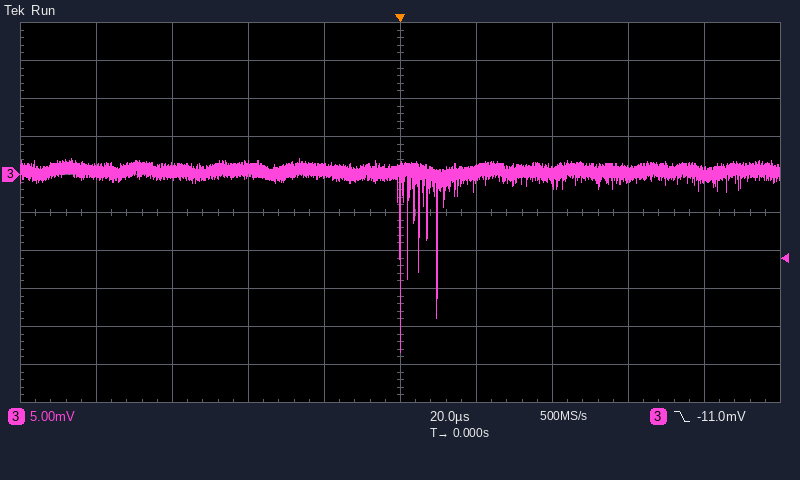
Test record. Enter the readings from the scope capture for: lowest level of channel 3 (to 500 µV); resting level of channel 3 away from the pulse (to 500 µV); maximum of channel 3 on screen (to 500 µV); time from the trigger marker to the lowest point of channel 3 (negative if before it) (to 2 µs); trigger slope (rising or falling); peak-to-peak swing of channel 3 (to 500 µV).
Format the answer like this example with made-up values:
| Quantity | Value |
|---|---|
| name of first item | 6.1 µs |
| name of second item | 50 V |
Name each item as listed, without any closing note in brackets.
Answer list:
| Quantity | Value |
|---|---|
| lowest level of channel 3 | -23.5 mV |
| resting level of channel 3 away from the pulse | 500 µV |
| maximum of channel 3 on screen | 2.0 mV |
| time from the trigger marker to the lowest point of channel 3 (negative if before it) | 0 µs |
| trigger slope | falling |
| peak-to-peak swing of channel 3 | 25.5 mV |
